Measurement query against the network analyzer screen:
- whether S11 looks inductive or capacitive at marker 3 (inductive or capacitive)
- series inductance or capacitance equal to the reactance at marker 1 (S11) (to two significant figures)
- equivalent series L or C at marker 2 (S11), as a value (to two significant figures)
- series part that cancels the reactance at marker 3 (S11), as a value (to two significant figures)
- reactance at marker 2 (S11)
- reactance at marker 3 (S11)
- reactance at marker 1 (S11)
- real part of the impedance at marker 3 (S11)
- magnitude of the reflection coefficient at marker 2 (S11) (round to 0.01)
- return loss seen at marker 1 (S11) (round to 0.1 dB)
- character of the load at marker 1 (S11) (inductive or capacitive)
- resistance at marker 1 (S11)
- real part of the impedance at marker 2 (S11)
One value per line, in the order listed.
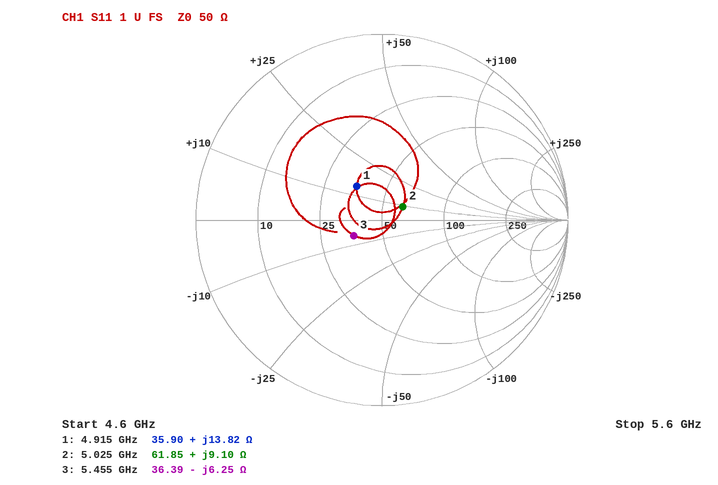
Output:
capacitive
450 pH
290 pH
180 pH
+9.10 Ω
-6.25 Ω
+13.82 Ω
36.39 Ω
0.13
12.9 dB
inductive
35.90 Ω
61.85 Ω
